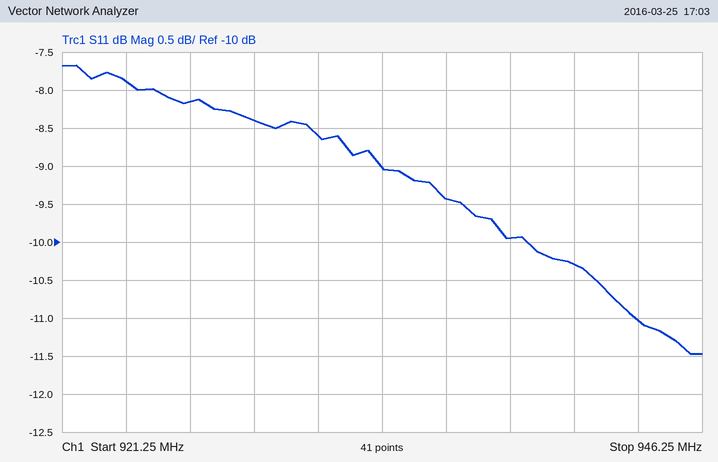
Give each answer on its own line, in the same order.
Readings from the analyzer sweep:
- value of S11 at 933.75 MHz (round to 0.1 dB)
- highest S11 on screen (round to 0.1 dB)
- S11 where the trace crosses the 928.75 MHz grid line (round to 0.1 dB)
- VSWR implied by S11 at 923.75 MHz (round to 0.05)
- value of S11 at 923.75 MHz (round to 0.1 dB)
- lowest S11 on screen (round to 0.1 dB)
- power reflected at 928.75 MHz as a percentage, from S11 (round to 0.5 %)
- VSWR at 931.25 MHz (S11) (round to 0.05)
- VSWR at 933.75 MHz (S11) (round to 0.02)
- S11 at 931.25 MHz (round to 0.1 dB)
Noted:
-9.0 dB
-7.7 dB
-8.4 dB
2.35
-7.9 dB
-11.5 dB
14.5 %
2.20
2.10
-8.6 dB
